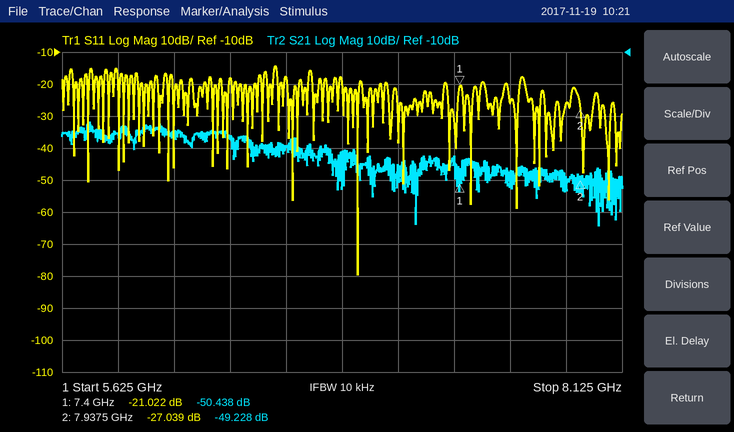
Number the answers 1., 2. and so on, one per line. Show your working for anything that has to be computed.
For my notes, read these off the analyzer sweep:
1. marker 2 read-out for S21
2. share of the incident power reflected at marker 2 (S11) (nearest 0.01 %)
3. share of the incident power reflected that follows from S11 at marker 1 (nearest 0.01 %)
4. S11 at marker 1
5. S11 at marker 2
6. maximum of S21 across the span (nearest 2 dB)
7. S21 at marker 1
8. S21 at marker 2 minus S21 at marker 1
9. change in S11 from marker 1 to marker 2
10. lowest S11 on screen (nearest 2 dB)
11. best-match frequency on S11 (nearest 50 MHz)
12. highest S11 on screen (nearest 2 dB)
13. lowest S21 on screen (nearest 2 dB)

1. -49.228 dB
2. 10^(-27.039/10) ≈ 0.20 %
3. 10^(-21.022/10) ≈ 0.79 %
4. -21.022 dB
5. -27.039 dB
6. -32 dB
7. -50.438 dB
8. -49.228 − (-50.438) = 1.210 dB
9. -27.039 − (-21.022) = -6.017 dB
10. -80 dB
11. 6.95 GHz
12. -14 dB
13. -64 dB
